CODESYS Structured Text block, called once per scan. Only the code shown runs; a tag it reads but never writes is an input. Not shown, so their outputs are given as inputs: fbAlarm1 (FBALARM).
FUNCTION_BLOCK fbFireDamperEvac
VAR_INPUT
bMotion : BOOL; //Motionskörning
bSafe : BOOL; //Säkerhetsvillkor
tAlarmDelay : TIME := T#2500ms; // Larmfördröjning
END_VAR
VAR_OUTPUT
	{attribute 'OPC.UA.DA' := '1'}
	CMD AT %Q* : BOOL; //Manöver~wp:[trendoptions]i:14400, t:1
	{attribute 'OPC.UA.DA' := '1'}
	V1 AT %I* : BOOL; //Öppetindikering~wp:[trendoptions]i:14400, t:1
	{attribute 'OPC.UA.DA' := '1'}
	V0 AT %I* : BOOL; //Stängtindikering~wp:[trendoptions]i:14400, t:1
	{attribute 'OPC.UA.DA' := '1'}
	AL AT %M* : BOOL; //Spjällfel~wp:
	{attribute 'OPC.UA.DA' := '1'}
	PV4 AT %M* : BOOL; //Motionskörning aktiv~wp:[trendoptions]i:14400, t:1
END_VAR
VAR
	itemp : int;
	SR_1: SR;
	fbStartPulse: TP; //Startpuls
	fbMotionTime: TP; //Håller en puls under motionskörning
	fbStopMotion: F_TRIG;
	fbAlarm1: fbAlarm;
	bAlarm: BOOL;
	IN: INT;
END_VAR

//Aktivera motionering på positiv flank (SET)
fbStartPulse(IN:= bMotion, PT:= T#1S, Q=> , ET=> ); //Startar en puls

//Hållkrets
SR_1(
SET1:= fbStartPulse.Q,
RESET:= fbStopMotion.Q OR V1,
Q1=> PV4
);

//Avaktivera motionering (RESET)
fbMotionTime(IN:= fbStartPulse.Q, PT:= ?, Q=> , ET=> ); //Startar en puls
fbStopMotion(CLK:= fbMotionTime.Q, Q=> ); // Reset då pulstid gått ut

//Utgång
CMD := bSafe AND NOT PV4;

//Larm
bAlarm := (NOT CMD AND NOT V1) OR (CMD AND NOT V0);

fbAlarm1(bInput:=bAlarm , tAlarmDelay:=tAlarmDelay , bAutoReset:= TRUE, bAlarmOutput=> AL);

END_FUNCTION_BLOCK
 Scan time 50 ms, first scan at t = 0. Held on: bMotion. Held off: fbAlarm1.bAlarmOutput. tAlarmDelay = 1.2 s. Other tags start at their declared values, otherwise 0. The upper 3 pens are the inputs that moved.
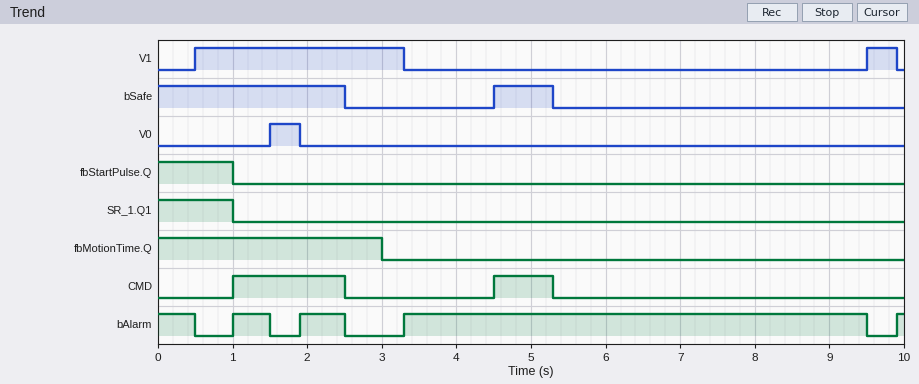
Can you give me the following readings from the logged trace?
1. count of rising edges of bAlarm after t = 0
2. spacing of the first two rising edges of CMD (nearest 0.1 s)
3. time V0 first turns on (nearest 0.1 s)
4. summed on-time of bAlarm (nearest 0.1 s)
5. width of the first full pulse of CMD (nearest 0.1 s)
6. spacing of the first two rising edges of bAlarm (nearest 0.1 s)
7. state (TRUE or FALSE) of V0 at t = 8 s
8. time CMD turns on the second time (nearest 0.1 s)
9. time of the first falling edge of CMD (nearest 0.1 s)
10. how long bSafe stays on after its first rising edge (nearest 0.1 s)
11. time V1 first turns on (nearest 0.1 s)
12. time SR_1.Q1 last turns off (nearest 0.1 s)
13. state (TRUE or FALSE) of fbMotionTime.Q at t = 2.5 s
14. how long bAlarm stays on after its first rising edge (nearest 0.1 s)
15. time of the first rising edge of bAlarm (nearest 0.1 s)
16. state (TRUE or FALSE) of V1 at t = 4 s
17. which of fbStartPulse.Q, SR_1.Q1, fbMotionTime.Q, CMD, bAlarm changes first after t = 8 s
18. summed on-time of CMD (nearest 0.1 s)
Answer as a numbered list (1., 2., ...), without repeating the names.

1. 4
2. 3.5 s
3. 1.5 s
4. 7.9 s
5. 1.5 s
6. 0.9 s
7. FALSE
8. 4.5 s
9. 2.5 s
10. 0.8 s
11. 0.5 s
12. 1.0 s
13. TRUE
14. 0.5 s
15. 1.0 s
16. FALSE
17. bAlarm
18. 2.3 s
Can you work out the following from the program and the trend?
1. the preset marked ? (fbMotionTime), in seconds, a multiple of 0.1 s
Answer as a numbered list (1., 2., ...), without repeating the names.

1. 3.0 s
